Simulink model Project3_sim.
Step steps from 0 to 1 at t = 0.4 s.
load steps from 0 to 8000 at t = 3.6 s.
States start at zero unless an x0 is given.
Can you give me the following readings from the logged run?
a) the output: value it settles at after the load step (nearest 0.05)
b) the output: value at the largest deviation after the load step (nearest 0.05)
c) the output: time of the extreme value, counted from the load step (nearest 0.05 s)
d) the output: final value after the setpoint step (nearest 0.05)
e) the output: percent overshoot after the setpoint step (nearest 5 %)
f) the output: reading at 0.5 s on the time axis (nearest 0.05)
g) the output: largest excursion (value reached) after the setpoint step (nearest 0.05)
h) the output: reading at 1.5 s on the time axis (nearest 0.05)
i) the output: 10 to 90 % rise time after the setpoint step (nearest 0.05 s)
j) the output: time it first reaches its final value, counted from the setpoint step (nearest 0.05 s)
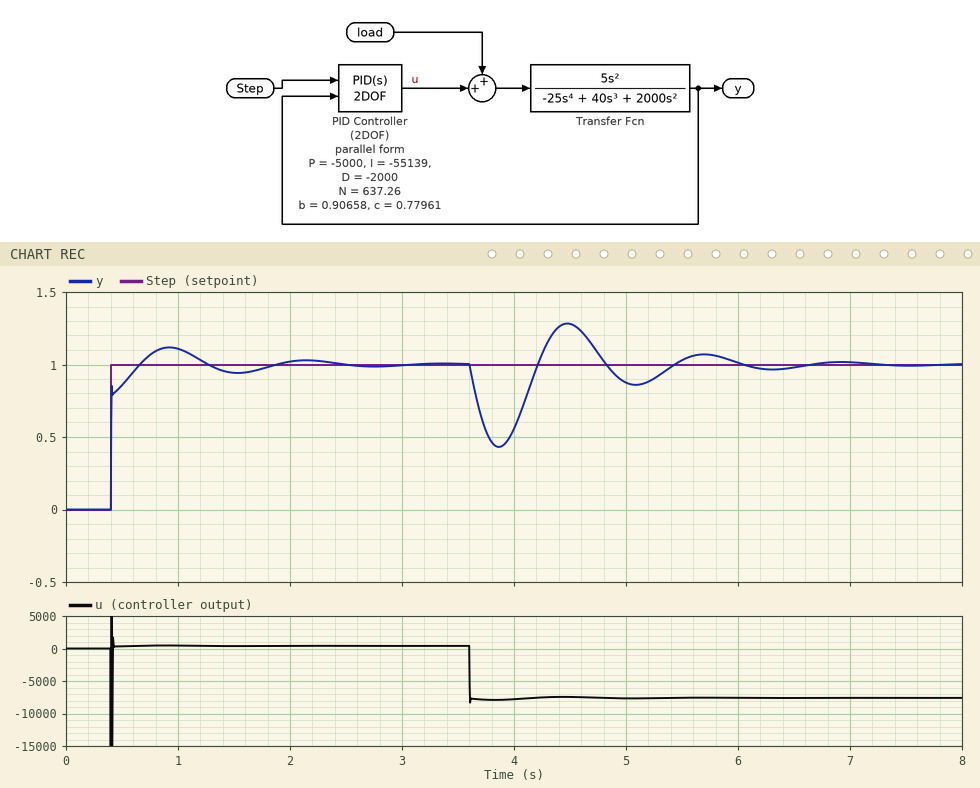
1.00
0.45
0.25 s
1.00
10 %
0.85
1.10
0.95
0.15 s
0.25 s
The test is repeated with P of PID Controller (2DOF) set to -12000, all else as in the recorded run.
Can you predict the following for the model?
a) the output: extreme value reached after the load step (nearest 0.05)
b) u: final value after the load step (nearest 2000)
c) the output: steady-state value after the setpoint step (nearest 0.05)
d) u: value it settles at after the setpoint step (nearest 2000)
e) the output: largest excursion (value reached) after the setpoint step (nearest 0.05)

0.60
-8000
1.00
0
1.05
